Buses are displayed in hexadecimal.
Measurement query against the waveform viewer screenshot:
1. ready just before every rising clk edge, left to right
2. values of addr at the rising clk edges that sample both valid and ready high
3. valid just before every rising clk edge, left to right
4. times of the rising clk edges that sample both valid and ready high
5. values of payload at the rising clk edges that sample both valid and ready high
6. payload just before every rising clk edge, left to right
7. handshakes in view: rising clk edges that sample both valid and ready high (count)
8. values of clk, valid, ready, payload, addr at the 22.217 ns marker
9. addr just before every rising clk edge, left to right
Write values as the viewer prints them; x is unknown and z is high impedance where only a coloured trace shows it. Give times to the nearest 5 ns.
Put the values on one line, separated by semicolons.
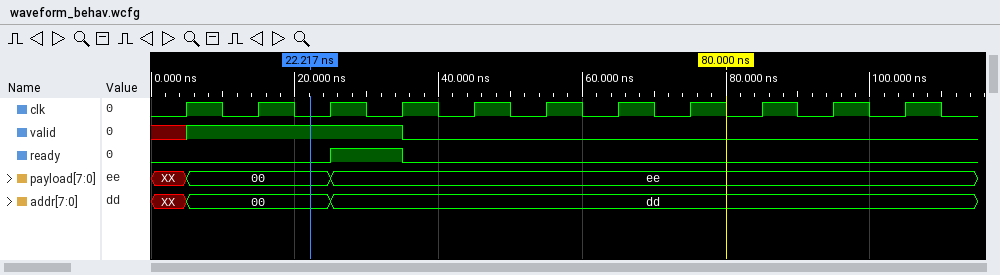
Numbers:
0 0 0 1 0 0 0 0 0 0 0; dd; x 1 1 1 0 0 0 0 0 0 0; 35 ns; ee; XX, 00, 00, ee, ee, ee, ee, ee, ee, ee, ee; 1; clk=0, valid=1, ready=0, payload=00, addr=00; XX, 00, 00, dd, dd, dd, dd, dd, dd, dd, dd
